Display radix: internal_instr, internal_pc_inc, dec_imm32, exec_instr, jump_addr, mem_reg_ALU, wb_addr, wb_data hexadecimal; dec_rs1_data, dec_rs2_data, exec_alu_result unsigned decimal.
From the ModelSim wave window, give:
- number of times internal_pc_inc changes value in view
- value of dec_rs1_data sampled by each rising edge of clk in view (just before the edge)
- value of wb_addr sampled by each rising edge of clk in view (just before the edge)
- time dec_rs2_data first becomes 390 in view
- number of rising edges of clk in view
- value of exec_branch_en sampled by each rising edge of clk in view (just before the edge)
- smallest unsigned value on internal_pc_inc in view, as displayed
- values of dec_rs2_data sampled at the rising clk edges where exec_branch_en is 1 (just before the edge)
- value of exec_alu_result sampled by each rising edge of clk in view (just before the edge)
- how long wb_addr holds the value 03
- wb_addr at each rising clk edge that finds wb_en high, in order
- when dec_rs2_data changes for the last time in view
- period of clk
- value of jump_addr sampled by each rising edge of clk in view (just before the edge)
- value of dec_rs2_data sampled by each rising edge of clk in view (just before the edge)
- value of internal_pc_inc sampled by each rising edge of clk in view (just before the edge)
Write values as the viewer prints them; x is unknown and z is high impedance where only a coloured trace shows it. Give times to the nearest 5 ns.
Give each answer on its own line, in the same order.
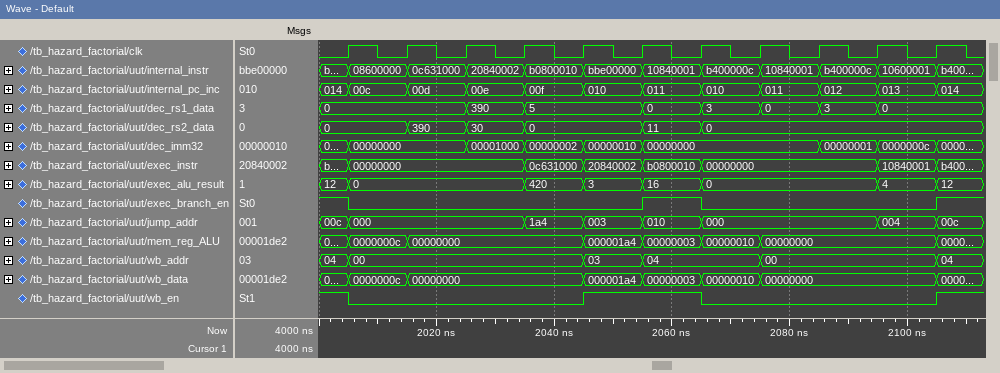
11
0, 0, 0, 390, 5, 5, 0, 3, 0, 3, 0
04, 00, 00, 00, 00, 03, 04, 04, 00, 00, 00
2015 ns
11
1 0 0 0 0 0 1 0 0 0 0
00c
0, 11
12, 0, 0, 0, 420, 3, 16, 0, 0, 0, 4
10 ns
04, 03, 04
2065 ns
10 ns
00c, 000, 000, 000, 1a4, 003, 010, 000, 000, 000, 004
0, 0, 390, 30, 0, 0, 11, 0, 0, 0, 0
014, 00c, 00d, 00e, 00f, 010, 011, 010, 011, 012, 013
